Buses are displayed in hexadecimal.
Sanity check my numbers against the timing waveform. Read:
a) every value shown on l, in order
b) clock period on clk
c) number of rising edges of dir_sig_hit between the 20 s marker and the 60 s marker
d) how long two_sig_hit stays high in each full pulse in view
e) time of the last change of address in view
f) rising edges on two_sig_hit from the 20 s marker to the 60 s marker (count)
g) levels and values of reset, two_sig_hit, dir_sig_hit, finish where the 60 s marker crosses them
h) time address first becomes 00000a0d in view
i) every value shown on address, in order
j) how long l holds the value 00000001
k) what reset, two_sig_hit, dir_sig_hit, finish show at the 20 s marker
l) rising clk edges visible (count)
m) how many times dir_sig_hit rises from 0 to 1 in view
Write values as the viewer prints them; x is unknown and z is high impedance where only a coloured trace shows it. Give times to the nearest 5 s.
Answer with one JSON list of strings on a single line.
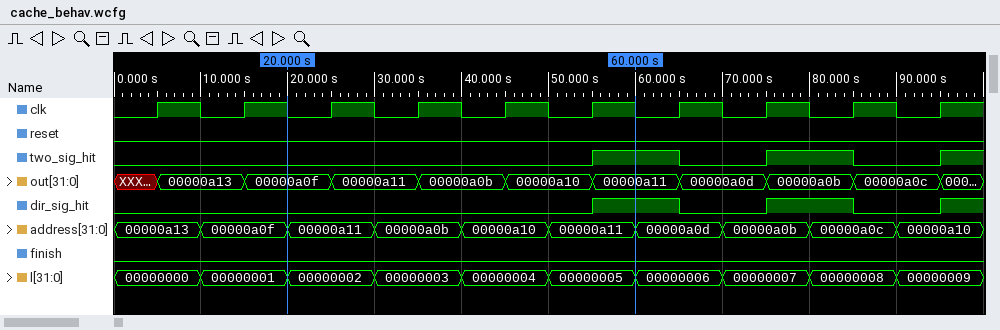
["00000000, 00000001, 00000002, 00000003, 00000004, 00000005, 00000006, 00000007, 00000008, 00000009", "10 s", "1", "10 s, 10 s", "90 s", "1", "reset=0, two_sig_hit=1, dir_sig_hit=1, finish=0", "60 s", "00000a13, 00000a0f, 00000a11, 00000a0b, 00000a10, 00000a11, 00000a0d, 00000a0b, 00000a0c, 00000a10", "10 s", "reset=0, two_sig_hit=0, dir_sig_hit=0, finish=0", "10", "3"]
